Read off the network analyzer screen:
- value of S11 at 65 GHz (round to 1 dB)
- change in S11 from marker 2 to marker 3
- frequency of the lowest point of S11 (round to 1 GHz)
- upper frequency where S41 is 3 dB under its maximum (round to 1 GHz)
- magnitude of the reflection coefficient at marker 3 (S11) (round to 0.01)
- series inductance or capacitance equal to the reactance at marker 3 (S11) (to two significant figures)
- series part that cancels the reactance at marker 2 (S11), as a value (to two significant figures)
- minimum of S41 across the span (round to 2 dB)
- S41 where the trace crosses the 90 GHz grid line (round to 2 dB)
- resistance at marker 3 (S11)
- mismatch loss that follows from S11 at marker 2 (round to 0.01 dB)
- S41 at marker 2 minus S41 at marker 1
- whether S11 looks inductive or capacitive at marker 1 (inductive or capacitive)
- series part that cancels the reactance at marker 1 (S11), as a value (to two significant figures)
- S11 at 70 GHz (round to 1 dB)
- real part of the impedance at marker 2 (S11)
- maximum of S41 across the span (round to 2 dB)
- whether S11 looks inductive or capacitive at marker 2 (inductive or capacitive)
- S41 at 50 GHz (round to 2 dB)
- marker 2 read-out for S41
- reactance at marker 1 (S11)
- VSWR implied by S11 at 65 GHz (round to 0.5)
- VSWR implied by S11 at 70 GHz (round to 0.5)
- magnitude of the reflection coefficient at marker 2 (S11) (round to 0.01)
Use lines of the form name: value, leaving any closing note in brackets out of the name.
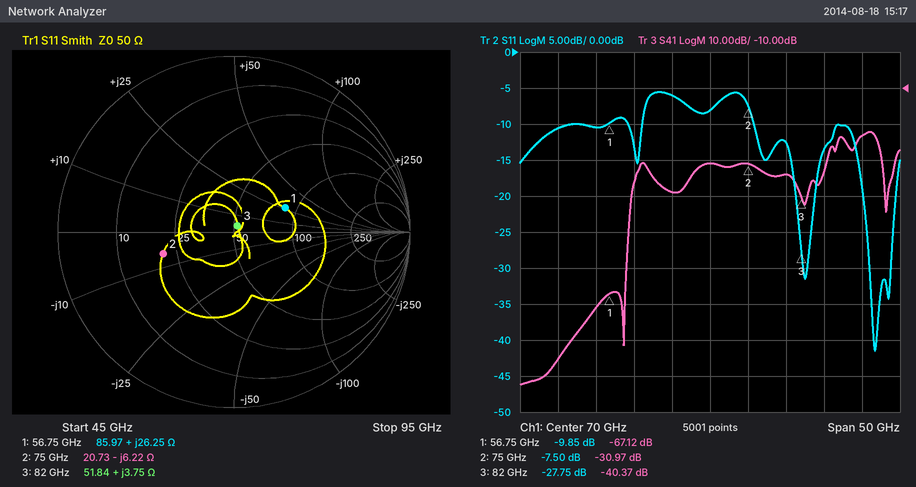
value of S11 at 65 GHz: -6 dB
change in S11 from marker 2 to marker 3: -20.25 dB
frequency of the lowest point of S11: 92 GHz
upper frequency where S41 is 3 dB under its maximum: 92 GHz
magnitude of the reflection coefficient at marker 3 (S11): 0.04
series inductance or capacitance equal to the reactance at marker 3 (S11): 7.3 pH
series part that cancels the reactance at marker 2 (S11), as a value: 13 pH
minimum of S41 across the span: -92 dB
S41 where the trace crosses the 90 GHz grid line: -24 dB
resistance at marker 3: 51.84 Ω
mismatch loss that follows from S11 at marker 2: 0.85 dB
S41 at marker 2 minus S41 at marker 1: 36.15 dB
whether S11 looks inductive or capacitive at marker 1: inductive
series part that cancels the reactance at marker 1 (S11), as a value: 110 fF
S11 at 70 GHz: -8 dB
real part of the impedance at marker 2: 20.73 Ω
maximum of S41 across the span: -22 dB
whether S11 looks inductive or capacitive at marker 2: capacitive
S41 at 50 GHz: -86 dB
marker 2 read-out for S41: -30.97 dB
reactance at marker 1: +26.25 Ω
VSWR implied by S11 at 65 GHz: 3.0
VSWR implied by S11 at 70 GHz: 2.5
magnitude of the reflection coefficient at marker 2 (S11): 0.42
